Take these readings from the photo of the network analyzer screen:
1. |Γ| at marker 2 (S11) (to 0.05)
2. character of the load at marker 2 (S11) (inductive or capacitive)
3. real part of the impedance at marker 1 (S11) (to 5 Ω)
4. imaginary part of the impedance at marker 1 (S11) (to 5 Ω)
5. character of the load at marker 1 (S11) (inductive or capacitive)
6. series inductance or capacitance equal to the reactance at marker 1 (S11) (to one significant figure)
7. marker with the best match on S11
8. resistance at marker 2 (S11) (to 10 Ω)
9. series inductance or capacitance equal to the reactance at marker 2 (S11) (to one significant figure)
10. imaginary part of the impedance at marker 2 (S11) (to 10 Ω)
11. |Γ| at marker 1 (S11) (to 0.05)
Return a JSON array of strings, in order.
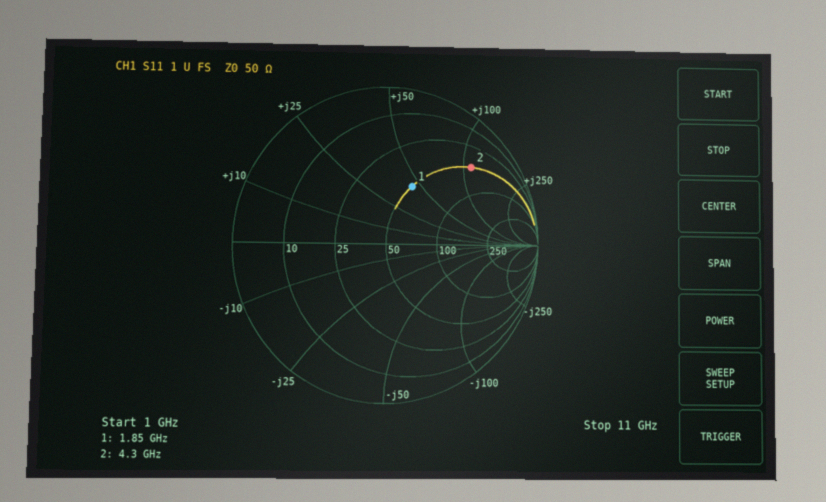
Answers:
["0.75", "inductive", "50 Ω", "+45 Ω", "inductive", "4 nH", "marker 1", "50 Ω", "4 nH", "+110 Ω", "0.40"]
